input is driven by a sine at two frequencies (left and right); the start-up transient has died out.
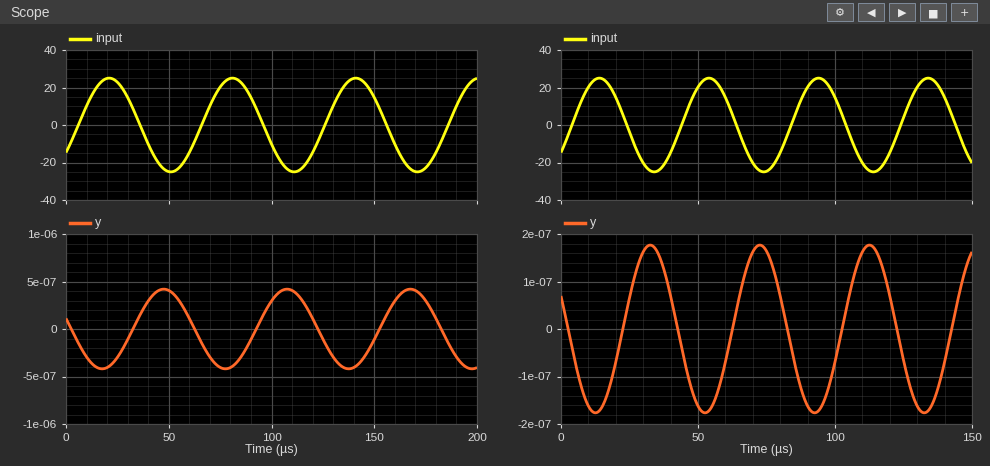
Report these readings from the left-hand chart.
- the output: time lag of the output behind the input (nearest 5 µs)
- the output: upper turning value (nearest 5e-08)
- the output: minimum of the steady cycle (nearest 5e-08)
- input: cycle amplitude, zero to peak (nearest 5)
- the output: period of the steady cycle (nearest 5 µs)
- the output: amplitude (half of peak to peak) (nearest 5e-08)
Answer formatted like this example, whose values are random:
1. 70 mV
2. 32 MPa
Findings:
1. 25 µs
2. 0.00000040
3. -0.00000040
4. 25
5. 60 µs
6. 0.00000040
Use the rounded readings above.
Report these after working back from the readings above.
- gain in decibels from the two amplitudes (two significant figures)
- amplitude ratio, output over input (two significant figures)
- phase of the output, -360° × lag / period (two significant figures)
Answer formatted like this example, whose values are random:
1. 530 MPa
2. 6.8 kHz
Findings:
1. -160 dB
2. 0.000000016
3. -150°
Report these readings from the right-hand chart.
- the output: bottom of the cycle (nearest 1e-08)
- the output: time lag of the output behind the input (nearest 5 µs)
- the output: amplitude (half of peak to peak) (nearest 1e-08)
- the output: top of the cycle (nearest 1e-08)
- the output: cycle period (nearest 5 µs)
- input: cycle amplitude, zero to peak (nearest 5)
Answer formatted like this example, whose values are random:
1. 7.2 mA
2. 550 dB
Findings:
1. -0.00000018
2. 20 µs
3. 0.00000018
4. 0.00000018
5. 40 µs
6. 25
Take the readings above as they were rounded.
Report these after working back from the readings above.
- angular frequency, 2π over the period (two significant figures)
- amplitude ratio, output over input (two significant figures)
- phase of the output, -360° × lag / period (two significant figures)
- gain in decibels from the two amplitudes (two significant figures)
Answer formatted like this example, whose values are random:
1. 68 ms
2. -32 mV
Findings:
1. 0.16 rad/µs
2. 0.0000000072
3. -180°
4. -160 dB
